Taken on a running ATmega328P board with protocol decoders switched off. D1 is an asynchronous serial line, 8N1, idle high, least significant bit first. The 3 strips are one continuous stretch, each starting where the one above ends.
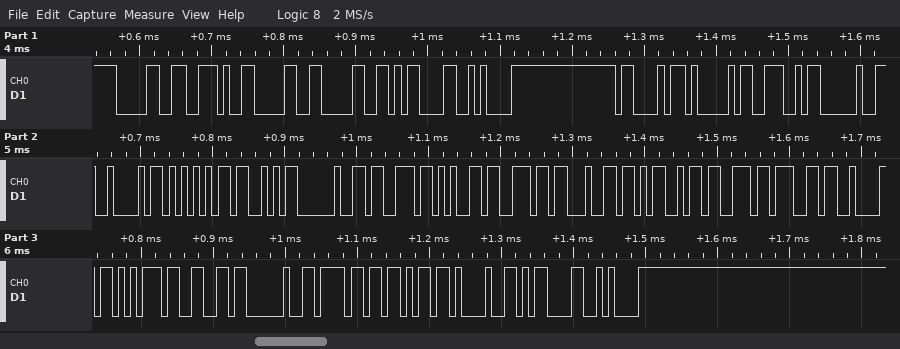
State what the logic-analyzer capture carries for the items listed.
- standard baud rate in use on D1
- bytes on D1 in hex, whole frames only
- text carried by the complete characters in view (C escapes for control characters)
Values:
115200 baud
0x30 0x2E 0x30 0x30 0x0D 0x0A 0x43 0x41 0x4E 0x20 0x42 0x55 0x53 0x20 0x73 0x65 0x6E 0x64 0x4D 0x73 0x67 0x42 0x75 0x66 0x20 0x6F 0x6B 0x21 0x0D 0x0A
"0.00\r\nCAN BUS sendMsgBuf ok!\r\n"
